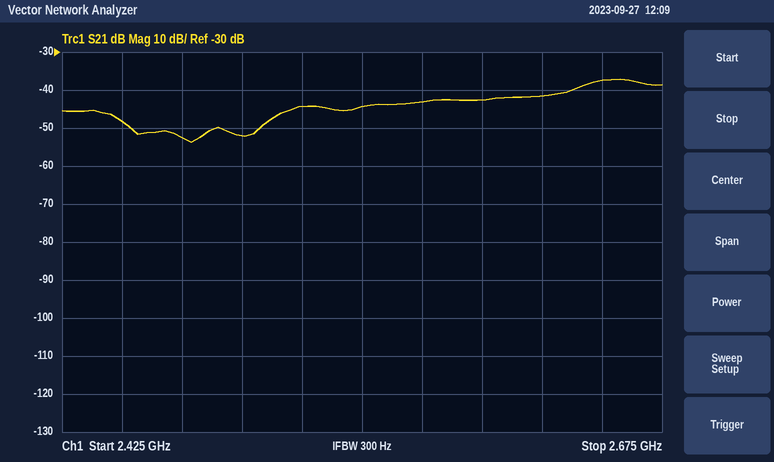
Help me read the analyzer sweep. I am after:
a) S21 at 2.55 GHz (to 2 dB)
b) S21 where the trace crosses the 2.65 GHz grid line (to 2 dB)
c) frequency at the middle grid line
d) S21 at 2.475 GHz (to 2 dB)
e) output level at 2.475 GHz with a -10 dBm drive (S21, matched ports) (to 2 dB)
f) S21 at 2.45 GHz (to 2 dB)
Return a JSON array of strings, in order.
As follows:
["-44 dB", "-38 dB", "2.55 GHz", "-52 dB", "-62 dBm", "-48 dB"]
